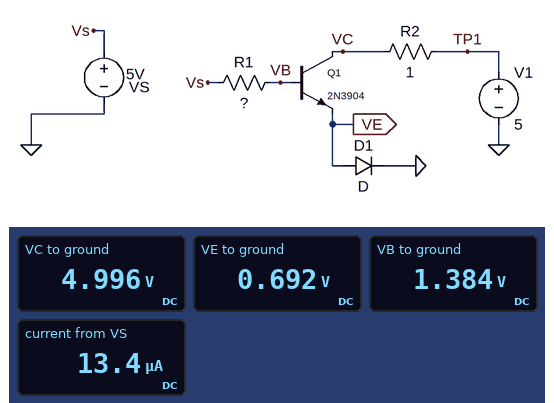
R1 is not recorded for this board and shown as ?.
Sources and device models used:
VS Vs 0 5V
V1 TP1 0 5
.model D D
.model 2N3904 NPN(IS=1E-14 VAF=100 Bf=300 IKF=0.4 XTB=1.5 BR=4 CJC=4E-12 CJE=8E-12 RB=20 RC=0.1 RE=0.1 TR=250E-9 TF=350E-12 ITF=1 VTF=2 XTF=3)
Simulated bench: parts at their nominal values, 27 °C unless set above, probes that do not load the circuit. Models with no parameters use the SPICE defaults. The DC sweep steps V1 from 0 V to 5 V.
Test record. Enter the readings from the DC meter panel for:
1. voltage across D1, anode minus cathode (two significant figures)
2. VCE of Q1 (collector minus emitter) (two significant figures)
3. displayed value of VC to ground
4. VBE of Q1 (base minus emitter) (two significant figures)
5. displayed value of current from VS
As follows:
690 mV
4.3 V
4.996 V
690 mV
13.4 µA
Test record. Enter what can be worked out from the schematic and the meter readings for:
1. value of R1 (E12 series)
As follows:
270 kΩ
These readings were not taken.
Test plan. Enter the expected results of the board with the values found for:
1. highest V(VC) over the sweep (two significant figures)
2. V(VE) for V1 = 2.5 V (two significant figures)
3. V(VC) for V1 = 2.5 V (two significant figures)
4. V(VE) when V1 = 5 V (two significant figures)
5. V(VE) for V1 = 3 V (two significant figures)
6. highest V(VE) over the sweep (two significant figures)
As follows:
5.0 V
690 mV
2.5 V
690 mV
690 mV
690 mV
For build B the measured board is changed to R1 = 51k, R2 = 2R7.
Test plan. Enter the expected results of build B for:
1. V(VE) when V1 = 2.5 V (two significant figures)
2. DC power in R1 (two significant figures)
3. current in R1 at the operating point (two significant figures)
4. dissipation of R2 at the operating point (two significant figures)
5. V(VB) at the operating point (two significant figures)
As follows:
730 mV
240 µW
69 µA
1.1 mW
1.5 V
